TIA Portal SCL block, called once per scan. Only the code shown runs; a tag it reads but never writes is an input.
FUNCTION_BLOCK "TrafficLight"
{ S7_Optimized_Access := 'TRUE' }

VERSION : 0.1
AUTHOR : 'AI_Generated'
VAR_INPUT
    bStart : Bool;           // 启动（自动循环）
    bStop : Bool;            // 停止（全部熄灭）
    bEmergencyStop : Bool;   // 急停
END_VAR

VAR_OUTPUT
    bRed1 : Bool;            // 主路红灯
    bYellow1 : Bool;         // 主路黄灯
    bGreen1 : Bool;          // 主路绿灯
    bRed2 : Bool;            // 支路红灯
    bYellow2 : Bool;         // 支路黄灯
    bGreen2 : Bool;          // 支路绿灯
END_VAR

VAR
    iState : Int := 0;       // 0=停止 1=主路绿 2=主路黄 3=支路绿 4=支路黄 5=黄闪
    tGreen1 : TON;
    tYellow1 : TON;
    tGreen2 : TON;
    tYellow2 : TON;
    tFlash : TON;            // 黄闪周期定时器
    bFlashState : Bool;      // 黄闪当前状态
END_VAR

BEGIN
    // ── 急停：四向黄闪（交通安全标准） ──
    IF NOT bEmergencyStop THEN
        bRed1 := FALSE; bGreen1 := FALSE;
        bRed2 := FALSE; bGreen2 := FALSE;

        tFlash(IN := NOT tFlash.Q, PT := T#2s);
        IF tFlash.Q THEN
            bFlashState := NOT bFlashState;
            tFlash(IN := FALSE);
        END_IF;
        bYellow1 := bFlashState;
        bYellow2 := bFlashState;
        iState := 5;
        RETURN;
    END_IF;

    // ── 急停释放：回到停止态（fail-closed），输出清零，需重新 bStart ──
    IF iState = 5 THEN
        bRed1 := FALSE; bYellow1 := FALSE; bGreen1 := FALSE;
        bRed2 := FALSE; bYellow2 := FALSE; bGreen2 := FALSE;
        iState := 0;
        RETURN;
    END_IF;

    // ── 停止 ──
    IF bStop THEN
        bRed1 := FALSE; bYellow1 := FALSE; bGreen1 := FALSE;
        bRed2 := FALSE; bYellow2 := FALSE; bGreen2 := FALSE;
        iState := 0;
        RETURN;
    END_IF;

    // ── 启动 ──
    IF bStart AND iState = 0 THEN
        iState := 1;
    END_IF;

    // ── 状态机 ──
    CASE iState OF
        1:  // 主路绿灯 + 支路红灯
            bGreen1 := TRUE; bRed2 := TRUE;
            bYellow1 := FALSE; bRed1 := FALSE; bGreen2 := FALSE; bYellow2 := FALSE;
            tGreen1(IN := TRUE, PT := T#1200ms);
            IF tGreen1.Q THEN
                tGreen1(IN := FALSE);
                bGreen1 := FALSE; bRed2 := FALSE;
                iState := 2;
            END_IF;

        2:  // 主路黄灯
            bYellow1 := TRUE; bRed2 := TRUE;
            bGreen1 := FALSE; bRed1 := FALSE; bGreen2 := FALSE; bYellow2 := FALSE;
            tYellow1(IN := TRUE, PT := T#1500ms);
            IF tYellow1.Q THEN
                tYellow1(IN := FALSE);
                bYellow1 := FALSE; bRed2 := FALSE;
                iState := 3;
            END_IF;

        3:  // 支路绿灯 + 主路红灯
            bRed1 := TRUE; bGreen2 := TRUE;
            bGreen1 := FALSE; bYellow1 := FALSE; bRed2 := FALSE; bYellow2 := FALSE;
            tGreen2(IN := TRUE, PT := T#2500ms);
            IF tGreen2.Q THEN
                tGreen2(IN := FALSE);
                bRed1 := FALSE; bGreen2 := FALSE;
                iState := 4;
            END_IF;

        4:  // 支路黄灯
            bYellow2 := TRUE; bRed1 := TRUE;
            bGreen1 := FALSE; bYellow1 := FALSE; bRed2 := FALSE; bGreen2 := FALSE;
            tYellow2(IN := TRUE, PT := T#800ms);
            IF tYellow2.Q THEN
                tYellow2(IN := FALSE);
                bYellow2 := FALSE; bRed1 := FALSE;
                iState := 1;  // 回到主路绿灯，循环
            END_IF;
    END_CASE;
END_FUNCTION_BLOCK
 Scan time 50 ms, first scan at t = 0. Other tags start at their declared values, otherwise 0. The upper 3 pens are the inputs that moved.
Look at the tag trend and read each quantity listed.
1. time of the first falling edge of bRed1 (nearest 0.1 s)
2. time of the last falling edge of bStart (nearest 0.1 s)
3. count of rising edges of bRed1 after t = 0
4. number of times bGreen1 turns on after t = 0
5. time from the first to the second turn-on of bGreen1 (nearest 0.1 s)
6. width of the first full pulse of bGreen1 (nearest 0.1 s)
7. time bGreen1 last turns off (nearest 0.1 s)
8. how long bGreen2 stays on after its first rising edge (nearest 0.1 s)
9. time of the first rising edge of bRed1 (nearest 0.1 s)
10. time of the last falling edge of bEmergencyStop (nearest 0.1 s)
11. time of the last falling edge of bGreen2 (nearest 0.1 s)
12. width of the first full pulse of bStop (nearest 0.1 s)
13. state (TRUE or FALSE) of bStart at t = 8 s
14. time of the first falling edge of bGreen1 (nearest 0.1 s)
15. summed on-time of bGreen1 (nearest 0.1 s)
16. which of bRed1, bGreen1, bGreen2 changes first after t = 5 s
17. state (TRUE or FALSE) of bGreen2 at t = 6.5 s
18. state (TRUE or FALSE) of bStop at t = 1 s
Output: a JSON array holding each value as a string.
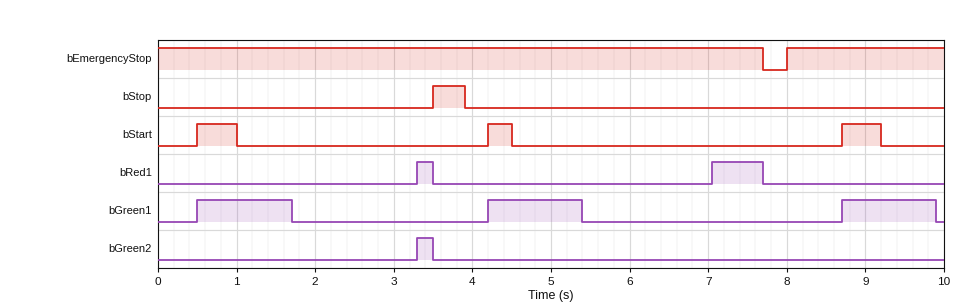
["3.5 s", "9.2 s", "2", "3", "3.7 s", "1.2 s", "9.9 s", "0.2 s", "3.3 s", "7.7 s", "3.5 s", "0.4 s", "FALSE", "1.7 s", "3.6 s", "bGreen1", "FALSE", "FALSE"]
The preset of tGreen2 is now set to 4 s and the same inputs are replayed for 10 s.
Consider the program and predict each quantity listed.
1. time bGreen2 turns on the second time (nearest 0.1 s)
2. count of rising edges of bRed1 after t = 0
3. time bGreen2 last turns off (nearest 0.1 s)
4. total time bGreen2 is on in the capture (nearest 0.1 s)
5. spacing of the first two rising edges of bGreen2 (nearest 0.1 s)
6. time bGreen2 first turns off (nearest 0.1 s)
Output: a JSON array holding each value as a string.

["7.0 s", "3", "7.3 s", "0.5 s", "3.7 s", "3.5 s"]
